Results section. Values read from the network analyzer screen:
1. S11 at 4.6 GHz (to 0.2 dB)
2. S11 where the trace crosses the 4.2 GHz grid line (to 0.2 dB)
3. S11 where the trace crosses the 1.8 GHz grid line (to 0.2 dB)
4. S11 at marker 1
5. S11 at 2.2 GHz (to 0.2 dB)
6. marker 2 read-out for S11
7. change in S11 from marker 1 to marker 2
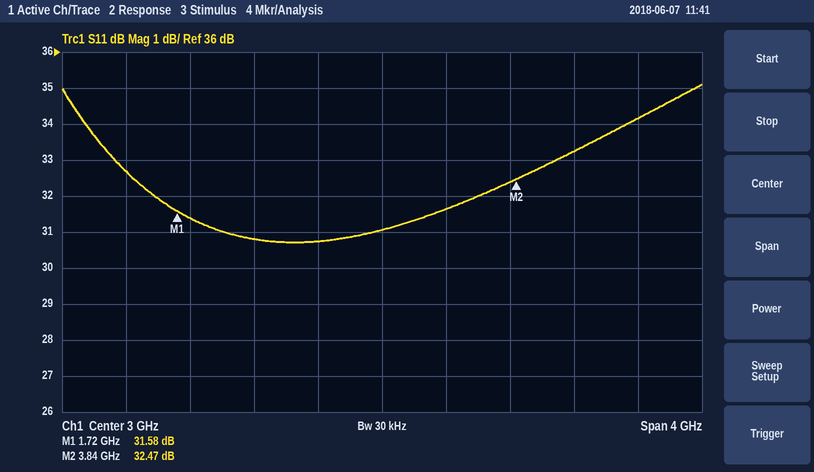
34.2 dB
33.2 dB
31.4 dB
31.58 dB
30.8 dB
32.47 dB
0.89 dB
